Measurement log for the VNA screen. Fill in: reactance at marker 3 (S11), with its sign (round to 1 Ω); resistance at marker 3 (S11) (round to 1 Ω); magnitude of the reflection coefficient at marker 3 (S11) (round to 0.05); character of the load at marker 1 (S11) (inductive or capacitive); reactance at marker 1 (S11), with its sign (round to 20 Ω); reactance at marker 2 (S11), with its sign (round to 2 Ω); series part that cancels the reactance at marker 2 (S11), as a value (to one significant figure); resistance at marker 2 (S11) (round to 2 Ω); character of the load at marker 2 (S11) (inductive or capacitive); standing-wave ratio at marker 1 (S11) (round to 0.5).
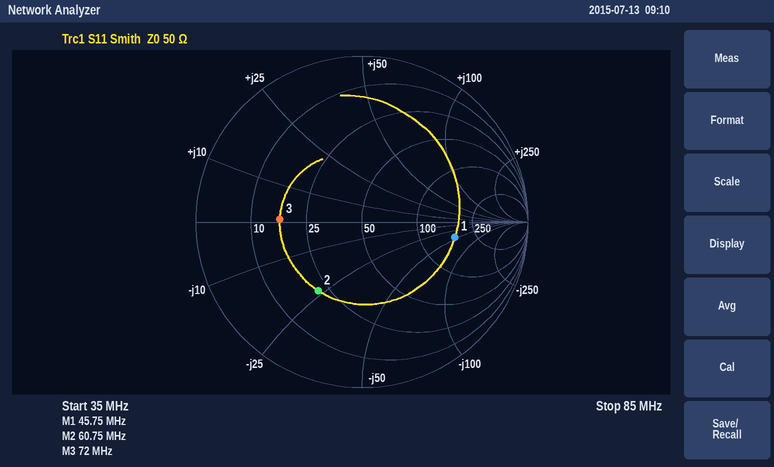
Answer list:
+1 Ω
17 Ω
0.50
capacitive
-40 Ω
-24 Ω
60 nH
22 Ω
capacitive
3.5
